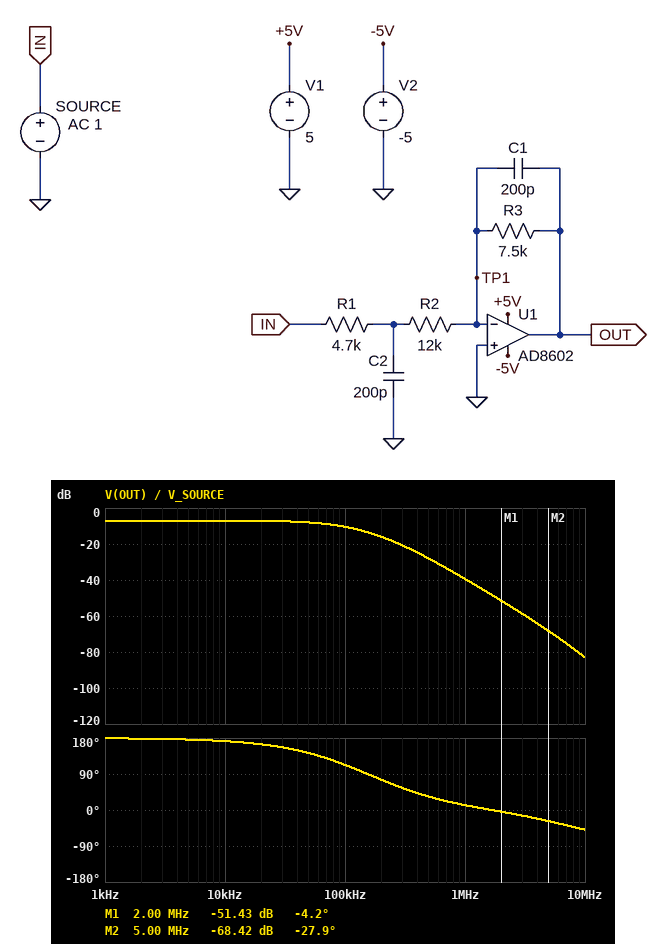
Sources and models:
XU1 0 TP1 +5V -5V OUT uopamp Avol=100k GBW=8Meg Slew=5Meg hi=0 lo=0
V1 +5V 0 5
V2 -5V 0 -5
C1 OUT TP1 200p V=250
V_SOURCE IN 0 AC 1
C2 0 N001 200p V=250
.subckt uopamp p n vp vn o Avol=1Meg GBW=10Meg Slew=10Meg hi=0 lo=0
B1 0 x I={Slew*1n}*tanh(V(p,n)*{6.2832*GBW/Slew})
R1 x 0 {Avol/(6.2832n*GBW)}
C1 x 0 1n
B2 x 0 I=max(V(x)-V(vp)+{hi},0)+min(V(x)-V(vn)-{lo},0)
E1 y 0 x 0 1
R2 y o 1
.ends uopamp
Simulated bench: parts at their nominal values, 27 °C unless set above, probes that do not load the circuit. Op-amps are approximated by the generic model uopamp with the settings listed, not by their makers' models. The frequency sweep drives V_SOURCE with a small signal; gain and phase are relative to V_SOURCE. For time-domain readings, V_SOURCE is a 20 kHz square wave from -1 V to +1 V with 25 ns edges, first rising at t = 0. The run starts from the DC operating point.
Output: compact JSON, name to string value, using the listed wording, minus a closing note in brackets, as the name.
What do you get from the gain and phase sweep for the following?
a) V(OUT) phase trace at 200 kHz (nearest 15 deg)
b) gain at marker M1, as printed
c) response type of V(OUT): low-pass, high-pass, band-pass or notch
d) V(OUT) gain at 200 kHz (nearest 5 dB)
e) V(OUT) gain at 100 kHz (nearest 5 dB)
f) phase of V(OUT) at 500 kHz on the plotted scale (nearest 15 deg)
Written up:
{"V(OUT) phase trace at 200 kHz": "75 deg", "gain at marker M1, as printed": "-51.43 dB", "response type of V(OUT): low-pass, high-pass, band-pass or notch": "low-pass", "V(OUT) gain at 200 kHz": "-15 dB", "V(OUT) gain at 100 kHz": "-10 dB", "phase of V(OUT) at 500 kHz on the plotted scale": "30 deg"}
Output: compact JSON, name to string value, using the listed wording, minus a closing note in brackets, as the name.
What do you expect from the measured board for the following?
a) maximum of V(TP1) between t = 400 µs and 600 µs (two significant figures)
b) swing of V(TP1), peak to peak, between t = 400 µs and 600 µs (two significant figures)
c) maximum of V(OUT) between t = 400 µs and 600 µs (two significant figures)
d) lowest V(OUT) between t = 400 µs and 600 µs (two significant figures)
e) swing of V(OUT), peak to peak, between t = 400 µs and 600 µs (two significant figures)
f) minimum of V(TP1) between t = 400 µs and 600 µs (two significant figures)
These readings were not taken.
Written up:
{"maximum of V(TP1) between t = 400 µs and 600 µs": "6.2 mV", "swing of V(TP1), peak to peak, between t = 400 µs and 600 µs": "12 mV", "maximum of V(OUT) between t = 400 µs and 600 µs": "450 mV", "lowest V(OUT) between t = 400 µs and 600 µs": "-450 mV", "swing of V(OUT), peak to peak, between t = 400 µs and 600 µs": "900 mV", "minimum of V(TP1) between t = 400 µs and 600 µs": "-6.2 mV"}
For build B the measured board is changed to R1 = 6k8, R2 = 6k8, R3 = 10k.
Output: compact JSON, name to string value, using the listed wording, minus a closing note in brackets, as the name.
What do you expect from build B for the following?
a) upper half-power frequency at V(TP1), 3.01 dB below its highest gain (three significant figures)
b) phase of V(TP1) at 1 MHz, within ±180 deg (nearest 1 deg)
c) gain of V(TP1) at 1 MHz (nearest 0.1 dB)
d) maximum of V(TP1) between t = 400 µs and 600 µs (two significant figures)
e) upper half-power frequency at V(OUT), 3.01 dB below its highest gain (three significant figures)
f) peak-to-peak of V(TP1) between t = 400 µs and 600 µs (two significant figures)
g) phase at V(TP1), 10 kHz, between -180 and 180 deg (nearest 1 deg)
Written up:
{"upper half-power frequency at V(TP1), 3.01 dB below its highest gain": "361 kHz", "phase of V(TP1) at 1 MHz, within ±180 deg": "-79 deg", "gain of V(TP1) at 1 MHz": "-55.8 dB", "maximum of V(TP1) between t = 400 µs and 600 µs": "8.4 mV", "upper half-power frequency at V(OUT), 3.01 dB below its highest gain": "72.0 kHz", "peak-to-peak of V(TP1) between t = 400 µs and 600 µs": "17 mV", "phase at V(TP1), 10 kHz, between -180 and 180 deg": "80 deg"}
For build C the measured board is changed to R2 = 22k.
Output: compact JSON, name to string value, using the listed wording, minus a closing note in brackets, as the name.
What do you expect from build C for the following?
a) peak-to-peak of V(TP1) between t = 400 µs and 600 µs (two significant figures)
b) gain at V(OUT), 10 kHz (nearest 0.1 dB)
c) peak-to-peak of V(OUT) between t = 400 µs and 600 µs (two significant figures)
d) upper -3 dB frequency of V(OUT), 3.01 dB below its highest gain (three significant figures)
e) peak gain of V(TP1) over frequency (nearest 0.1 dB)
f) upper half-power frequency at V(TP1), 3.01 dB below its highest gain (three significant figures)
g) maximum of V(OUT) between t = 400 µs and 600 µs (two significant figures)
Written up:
{"peak-to-peak of V(TP1) between t = 400 µs and 600 µs": "7.4 mV", "gain at V(OUT), 10 kHz": "-11.1 dB", "peak-to-peak of V(OUT) between t = 400 µs and 600 µs": "560 mV", "upper -3 dB frequency of V(OUT), 3.01 dB below its highest gain": "87.9 kHz", "peak gain of V(TP1) over frequency": "-52.2 dB", "upper half-power frequency at V(TP1), 3.01 dB below its highest gain": "369 kHz", "maximum of V(OUT) between t = 400 µs and 600 µs": "280 mV"}
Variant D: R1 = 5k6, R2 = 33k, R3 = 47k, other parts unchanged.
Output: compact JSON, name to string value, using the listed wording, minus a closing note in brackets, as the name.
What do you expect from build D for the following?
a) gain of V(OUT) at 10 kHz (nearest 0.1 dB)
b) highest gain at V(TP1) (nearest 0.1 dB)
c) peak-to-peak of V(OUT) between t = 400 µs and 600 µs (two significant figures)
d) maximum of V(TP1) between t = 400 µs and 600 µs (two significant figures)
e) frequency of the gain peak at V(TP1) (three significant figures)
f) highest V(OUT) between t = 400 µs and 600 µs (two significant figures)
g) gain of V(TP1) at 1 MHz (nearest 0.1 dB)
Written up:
{"gain of V(OUT) at 10 kHz": "0.4 dB", "highest gain at V(TP1)": "-52.6 dB", "peak-to-peak of V(OUT) between t = 400 µs and 600 µs": "2.1 V", "maximum of V(TP1) between t = 400 µs and 600 µs": "3.7 mV", "frequency of the gain peak at V(TP1)": "53.0 kHz", "highest V(OUT) between t = 400 µs and 600 µs": "1.0 V", "gain of V(TP1) at 1 MHz": "-67.6 dB"}
